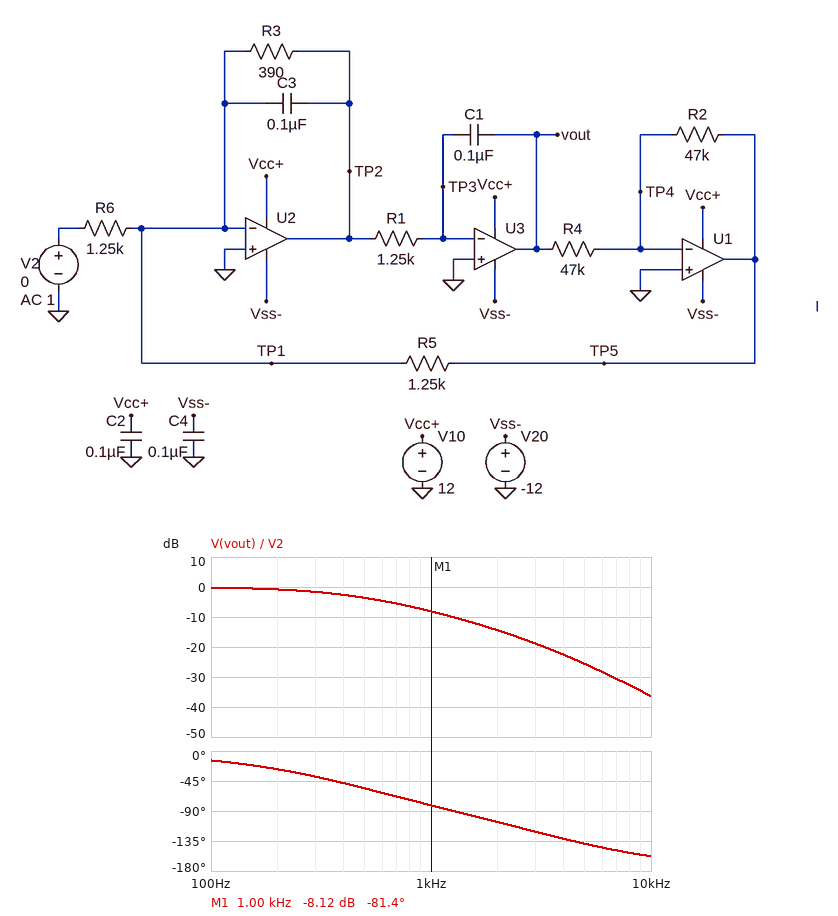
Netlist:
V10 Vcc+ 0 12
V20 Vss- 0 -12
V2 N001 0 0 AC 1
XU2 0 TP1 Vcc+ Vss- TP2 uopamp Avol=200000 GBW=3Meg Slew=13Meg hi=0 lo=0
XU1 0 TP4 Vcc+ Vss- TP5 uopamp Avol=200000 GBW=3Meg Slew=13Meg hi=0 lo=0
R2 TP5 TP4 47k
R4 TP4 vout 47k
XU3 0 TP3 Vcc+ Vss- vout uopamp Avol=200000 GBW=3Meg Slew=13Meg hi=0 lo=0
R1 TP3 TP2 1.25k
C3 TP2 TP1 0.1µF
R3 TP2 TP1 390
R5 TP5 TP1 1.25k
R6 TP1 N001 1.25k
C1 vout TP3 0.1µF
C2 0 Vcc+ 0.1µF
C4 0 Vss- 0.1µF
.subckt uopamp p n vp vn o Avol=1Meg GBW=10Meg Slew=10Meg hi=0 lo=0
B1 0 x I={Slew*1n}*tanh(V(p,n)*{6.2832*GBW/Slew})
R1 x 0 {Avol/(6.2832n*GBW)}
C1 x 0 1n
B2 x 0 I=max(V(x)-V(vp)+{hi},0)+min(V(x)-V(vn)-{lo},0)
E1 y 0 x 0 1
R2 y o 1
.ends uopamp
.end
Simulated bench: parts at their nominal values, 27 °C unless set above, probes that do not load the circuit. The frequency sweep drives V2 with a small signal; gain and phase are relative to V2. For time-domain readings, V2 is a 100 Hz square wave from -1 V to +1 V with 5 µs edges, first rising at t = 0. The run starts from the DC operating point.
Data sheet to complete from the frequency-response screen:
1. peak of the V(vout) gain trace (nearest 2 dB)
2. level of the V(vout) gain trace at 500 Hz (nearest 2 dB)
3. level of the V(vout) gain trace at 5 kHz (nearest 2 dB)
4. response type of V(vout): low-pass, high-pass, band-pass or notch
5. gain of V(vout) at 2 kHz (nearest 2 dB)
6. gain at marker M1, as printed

0 dB
-4 dB
-26 dB
low-pass
-14 dB
-8.12 dB
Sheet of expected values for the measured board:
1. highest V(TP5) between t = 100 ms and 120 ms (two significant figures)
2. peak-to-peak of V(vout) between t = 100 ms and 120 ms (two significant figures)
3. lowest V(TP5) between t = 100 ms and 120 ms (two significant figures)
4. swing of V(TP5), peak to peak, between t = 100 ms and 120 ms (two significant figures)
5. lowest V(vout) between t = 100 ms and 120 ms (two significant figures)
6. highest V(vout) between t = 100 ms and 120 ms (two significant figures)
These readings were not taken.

1.0 V
2.0 V
-1.0 V
2.0 V
-1.0 V
1.0 V
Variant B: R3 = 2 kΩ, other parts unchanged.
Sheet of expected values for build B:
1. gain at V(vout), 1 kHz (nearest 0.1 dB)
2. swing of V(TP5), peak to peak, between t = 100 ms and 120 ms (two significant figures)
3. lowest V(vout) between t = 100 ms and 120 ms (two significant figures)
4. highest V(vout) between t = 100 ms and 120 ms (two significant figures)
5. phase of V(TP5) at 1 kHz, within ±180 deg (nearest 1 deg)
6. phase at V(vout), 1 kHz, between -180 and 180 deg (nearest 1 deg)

4.1 dB
3.4 V
-1.7 V
1.7 V
128 deg
-52 deg
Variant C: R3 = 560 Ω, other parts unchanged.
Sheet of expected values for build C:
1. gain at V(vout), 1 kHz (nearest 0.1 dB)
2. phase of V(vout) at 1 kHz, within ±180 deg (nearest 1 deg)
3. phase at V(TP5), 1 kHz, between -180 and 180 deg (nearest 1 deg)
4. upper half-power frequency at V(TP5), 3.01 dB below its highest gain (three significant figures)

-5.1 dB
-78 deg
102 deg
703 Hz
